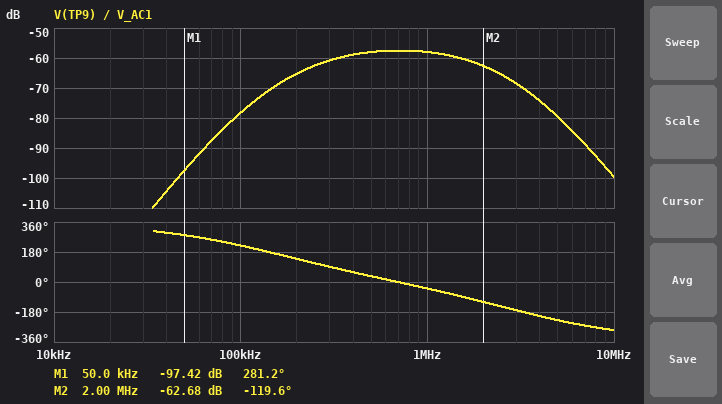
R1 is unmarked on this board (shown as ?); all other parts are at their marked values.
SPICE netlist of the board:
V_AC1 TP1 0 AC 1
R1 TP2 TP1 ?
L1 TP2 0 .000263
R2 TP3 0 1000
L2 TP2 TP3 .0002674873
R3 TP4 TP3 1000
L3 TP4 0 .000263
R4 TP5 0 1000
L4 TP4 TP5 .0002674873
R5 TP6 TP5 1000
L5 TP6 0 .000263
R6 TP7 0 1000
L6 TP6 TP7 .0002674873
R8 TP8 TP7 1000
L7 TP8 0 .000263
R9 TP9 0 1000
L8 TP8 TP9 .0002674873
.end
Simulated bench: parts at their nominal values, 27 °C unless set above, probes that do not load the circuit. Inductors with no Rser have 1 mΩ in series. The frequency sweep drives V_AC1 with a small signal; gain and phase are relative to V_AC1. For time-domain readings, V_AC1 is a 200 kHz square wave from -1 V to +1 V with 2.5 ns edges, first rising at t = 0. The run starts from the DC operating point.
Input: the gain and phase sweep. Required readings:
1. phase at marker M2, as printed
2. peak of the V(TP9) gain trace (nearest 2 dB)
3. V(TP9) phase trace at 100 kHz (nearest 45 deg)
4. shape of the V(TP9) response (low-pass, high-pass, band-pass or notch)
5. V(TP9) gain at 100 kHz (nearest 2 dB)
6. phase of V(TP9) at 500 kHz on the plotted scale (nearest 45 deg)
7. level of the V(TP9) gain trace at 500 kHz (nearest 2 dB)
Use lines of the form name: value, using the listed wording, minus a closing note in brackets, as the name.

phase at marker M2, as printed: -119.6 deg
peak of the V(TP9) gain trace: -58 dB
V(TP9) phase trace at 100 kHz: 225 deg
shape of the V(TP9) response: band-pass
V(TP9) gain at 100 kHz: -78 dB
phase of V(TP9) at 500 kHz on the plotted scale: 45 deg
level of the V(TP9) gain trace at 500 kHz: -58 dB
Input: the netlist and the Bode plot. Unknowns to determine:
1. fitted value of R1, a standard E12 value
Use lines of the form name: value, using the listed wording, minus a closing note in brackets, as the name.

fitted value of R1, a standard E12 value: 2.7 kΩ
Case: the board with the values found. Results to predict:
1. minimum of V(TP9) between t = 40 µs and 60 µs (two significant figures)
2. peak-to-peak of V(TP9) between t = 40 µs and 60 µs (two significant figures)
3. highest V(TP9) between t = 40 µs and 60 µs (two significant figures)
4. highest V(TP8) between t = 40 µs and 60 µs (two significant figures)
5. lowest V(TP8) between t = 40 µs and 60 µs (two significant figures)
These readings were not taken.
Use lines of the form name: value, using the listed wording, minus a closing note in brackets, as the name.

minimum of V(TP9) between t = 40 µs and 60 µs: -1.5 mV
peak-to-peak of V(TP9) between t = 40 µs and 60 µs: 3.0 mV
highest V(TP9) between t = 40 µs and 60 µs: 1.5 mV
highest V(TP8) between t = 40 µs and 60 µs: 3.3 mV
lowest V(TP8) between t = 40 µs and 60 µs: -3.3 mV
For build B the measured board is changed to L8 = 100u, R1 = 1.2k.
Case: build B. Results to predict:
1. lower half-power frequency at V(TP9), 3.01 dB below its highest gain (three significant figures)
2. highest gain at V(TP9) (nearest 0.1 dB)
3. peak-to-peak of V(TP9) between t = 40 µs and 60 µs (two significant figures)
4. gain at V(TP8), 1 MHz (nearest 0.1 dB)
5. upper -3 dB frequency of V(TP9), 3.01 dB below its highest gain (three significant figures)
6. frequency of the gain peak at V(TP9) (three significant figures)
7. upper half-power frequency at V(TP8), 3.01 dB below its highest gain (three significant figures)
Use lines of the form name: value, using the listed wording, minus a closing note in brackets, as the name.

lower half-power frequency at V(TP9), 3.01 dB below its highest gain: 326 kHz
highest gain at V(TP9): -49.4 dB
peak-to-peak of V(TP9) between t = 40 µs and 60 µs: 7.1 mV
gain at V(TP8), 1 MHz: -48.6 dB
upper -3 dB frequency of V(TP9), 3.01 dB below its highest gain: 1.50 MHz
frequency of the gain peak at V(TP9): 704 kHz
upper half-power frequency at V(TP8), 3.01 dB below its highest gain: 2.08 MHz
